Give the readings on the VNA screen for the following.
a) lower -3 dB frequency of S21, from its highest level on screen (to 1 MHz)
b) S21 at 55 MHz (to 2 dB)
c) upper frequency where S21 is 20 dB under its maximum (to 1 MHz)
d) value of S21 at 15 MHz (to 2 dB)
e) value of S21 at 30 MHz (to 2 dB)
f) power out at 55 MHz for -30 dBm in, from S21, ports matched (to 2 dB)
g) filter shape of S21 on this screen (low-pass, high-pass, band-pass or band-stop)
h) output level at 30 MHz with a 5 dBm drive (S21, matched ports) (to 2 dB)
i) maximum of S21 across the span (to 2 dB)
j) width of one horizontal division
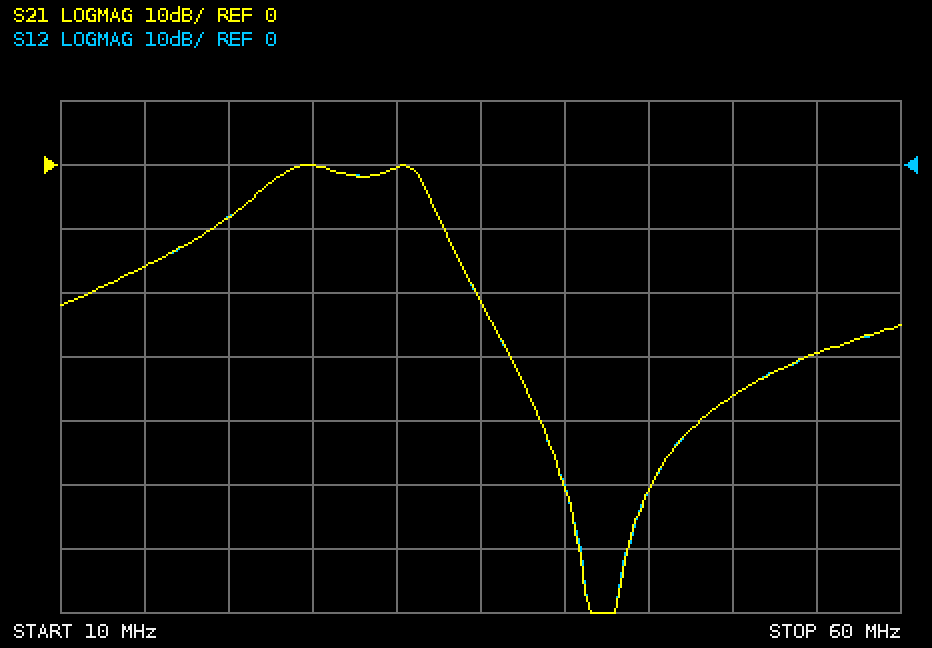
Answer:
22 MHz
-30 dB
35 MHz
-16 dB
0 dB
-60 dBm
band-pass
4 dBm
0 dB
5 MHz
